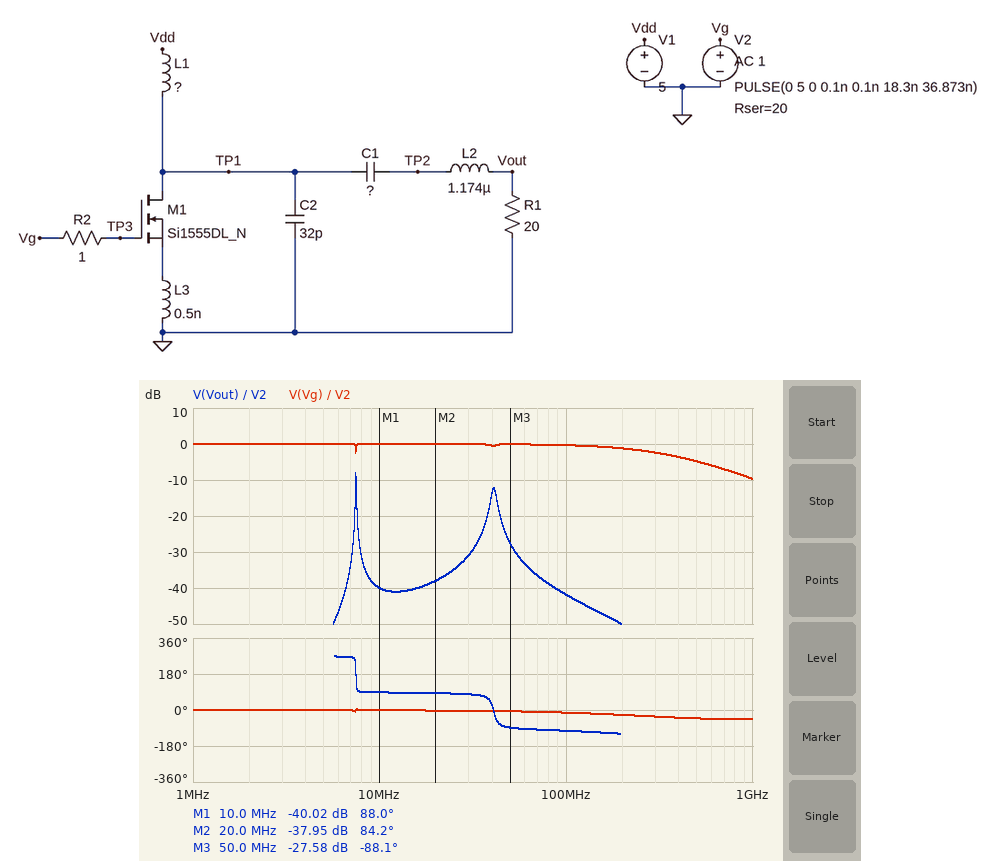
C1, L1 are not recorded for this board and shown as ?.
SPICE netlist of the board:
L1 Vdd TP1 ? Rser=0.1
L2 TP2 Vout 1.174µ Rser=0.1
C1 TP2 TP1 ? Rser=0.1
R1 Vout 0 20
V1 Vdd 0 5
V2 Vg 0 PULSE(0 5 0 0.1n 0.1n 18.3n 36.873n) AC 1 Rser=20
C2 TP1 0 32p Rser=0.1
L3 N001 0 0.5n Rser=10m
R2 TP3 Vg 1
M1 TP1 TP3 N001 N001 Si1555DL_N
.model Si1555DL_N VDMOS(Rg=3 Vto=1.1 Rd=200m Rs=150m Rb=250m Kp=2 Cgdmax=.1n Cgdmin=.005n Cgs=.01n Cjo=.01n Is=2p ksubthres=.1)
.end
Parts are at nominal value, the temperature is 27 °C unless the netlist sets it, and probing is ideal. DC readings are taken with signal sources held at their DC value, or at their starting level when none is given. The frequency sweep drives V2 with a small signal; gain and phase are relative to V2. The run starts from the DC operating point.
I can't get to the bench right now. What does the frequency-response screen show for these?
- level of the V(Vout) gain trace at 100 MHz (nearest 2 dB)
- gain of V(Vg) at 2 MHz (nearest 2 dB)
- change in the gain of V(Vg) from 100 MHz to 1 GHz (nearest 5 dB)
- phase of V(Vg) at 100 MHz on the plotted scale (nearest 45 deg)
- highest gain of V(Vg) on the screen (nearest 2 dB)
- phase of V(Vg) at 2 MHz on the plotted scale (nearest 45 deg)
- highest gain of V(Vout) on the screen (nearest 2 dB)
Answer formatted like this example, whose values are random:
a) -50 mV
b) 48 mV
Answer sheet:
a) -42 dB
b) 0 dB
c) -10 dB
d) 0 deg
e) 0 dB
f) 0 deg
g) -8 dB
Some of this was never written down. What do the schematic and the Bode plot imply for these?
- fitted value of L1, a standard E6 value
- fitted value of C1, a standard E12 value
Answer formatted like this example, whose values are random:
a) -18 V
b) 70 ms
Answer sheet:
a) 6.8 µH
b) 18 pF
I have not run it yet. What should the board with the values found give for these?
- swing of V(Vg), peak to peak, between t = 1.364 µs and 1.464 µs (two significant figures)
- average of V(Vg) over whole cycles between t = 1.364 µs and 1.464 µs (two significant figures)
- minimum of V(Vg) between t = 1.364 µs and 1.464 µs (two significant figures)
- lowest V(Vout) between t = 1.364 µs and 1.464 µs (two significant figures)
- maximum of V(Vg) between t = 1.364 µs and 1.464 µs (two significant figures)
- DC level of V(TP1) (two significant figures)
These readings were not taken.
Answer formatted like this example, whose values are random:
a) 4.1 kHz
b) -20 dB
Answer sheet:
a) 4.6 V
b) 2.5 V
c) 370 mV
d) -1.7 V
e) 5.0 V
f) 5.0 V
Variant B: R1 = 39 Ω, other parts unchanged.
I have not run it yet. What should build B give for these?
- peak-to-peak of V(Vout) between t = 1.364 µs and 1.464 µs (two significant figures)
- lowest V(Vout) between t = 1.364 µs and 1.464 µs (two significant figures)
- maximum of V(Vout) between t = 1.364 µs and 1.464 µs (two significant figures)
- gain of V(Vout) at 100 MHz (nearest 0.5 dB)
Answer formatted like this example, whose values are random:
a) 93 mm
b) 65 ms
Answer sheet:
a) 5.8 V
b) -3.3 V
c) 2.6 V
d) -36.0 dB
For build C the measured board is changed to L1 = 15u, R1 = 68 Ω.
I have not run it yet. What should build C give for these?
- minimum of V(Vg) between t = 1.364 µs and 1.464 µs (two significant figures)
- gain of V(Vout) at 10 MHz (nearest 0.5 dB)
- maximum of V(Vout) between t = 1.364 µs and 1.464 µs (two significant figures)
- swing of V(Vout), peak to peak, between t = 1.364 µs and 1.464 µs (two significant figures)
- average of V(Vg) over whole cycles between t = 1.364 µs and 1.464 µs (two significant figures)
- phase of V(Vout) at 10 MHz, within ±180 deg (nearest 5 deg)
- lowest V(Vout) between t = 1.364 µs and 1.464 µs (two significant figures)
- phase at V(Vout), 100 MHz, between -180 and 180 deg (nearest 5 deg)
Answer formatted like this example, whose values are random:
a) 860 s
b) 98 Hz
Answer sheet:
a) 310 mV
b) -34.0 dB
c) 3.5 V
d) 8.8 V
e) 2.5 V
f) 85 deg
g) -5.3 V
h) -100 deg
